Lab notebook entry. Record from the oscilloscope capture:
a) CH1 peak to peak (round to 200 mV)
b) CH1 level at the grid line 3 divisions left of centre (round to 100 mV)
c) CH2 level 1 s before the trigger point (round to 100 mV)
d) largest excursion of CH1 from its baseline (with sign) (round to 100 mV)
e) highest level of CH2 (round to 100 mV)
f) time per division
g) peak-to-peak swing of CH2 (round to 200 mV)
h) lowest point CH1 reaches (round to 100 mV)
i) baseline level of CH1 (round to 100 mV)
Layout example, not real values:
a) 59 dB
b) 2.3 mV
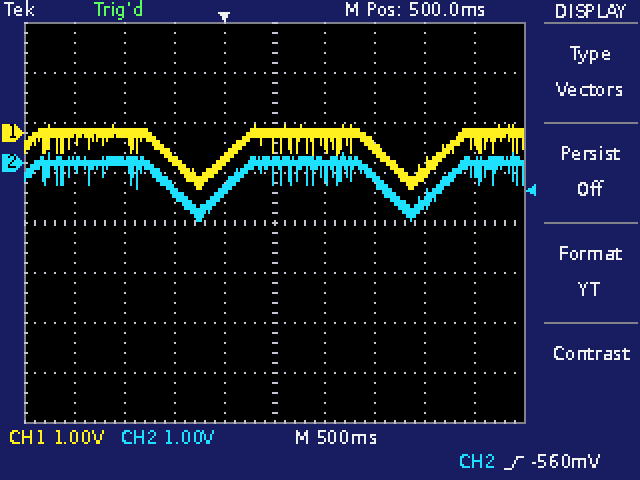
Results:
a) 1.2 V
b) 0.0 V
c) 0.0 V
d) -1.1 V
e) 200 mV
f) 500 ms
g) 1.4 V
h) -1.1 V
i) 0.0 V
